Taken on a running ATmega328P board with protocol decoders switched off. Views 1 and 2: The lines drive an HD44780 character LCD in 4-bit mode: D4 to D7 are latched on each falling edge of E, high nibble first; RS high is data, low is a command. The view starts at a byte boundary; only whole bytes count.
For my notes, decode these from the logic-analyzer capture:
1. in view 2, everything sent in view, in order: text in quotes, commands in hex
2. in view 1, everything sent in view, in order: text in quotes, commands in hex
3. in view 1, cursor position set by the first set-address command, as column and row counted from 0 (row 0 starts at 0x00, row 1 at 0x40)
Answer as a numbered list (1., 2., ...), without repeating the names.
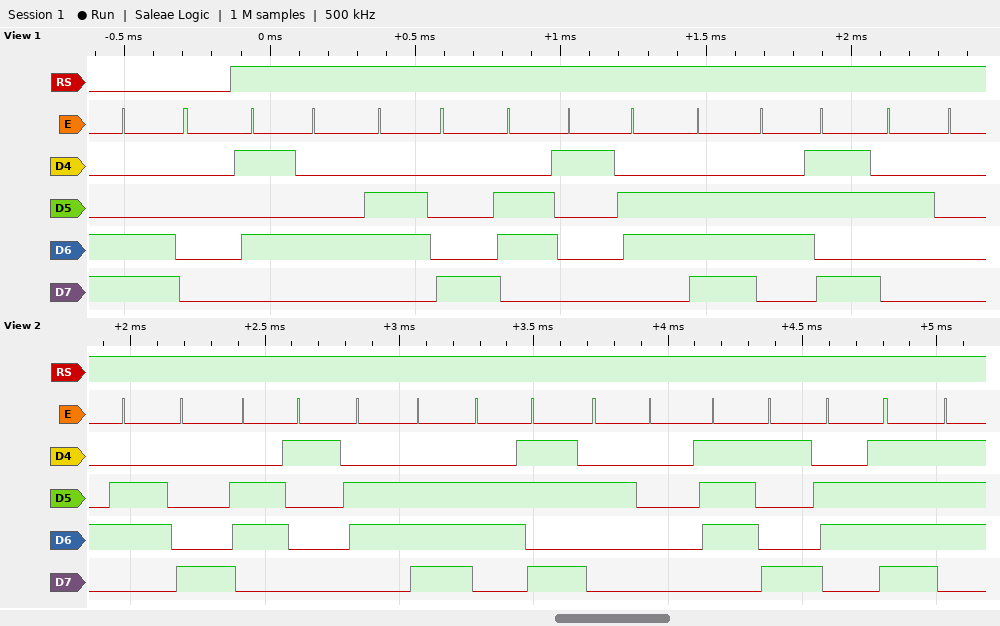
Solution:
1. "hank yo"
2. 0xC0 "Thank "
3. column 0, row 1
